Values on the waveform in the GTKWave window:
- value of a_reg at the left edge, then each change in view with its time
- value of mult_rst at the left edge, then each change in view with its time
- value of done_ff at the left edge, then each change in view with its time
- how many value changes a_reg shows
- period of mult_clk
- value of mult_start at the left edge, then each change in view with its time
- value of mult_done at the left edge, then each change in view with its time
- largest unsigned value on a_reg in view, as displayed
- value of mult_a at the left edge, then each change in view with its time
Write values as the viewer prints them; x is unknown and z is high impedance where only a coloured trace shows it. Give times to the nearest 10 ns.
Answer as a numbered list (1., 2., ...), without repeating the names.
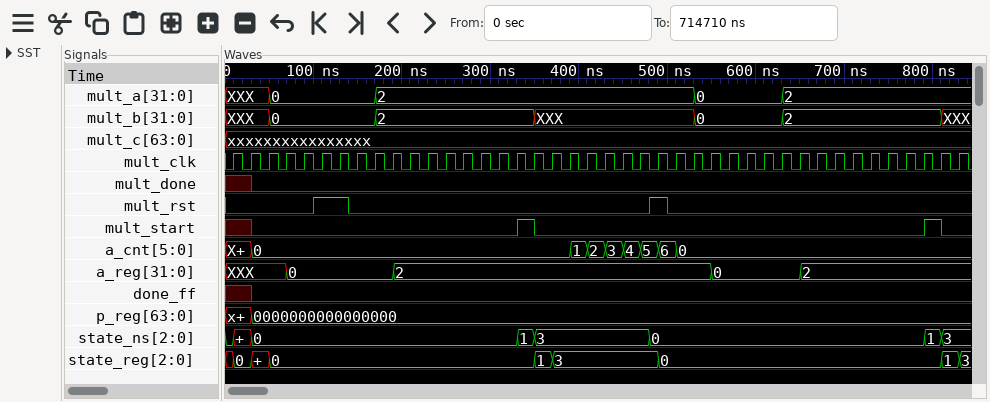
1. XXX, 0 at 70 ns, 2 at 190 ns, 0 at 550 ns, 2 at 650 ns
2. 0, 1 at 100 ns, 0 at 140 ns, 1 at 480 ns, 0 at 500 ns
3. x, 0 at 30 ns
4. 4
5. 20 ns
6. x, 0 at 30 ns, 1 at 330 ns, 0 at 350 ns, 1 at 790 ns, 0 at 810 ns
7. x, 0 at 30 ns
8. 2
9. XXX, 0 at 50 ns, 2 at 170 ns, 0 at 530 ns, 2 at 630 ns
